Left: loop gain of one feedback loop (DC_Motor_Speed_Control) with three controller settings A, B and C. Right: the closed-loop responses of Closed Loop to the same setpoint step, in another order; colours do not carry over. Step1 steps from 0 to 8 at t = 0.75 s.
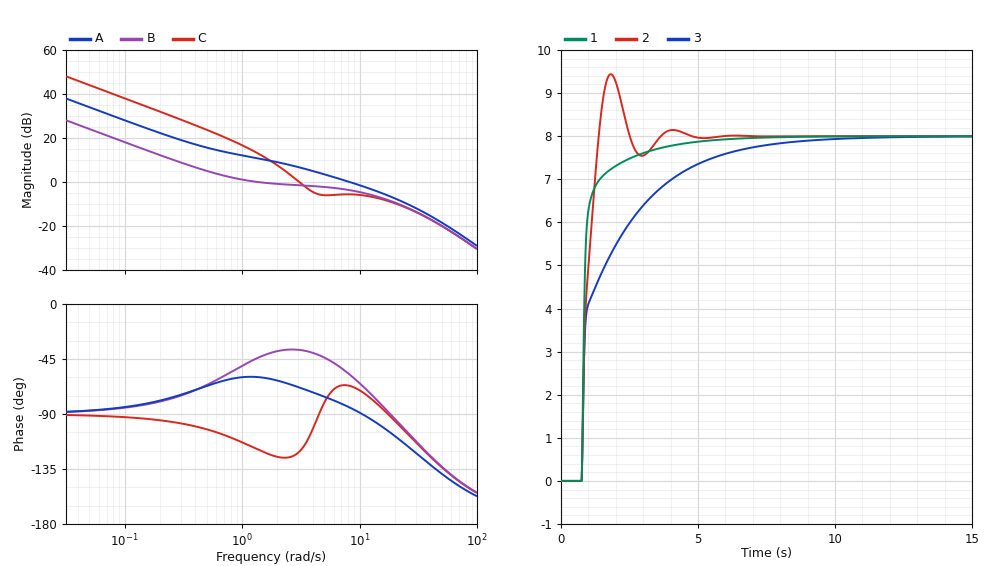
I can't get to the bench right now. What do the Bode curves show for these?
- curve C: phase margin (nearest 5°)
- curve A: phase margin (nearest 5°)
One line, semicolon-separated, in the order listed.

60°; 95°
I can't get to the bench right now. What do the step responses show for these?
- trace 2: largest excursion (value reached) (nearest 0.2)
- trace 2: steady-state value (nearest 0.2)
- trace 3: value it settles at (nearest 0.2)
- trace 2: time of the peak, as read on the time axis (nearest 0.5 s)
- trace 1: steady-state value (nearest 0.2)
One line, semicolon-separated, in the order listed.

9.4; 8.0; 8.0; 2.0 s; 8.0
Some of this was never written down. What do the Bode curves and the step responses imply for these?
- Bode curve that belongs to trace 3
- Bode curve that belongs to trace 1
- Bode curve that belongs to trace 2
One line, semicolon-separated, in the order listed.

B; A; C
